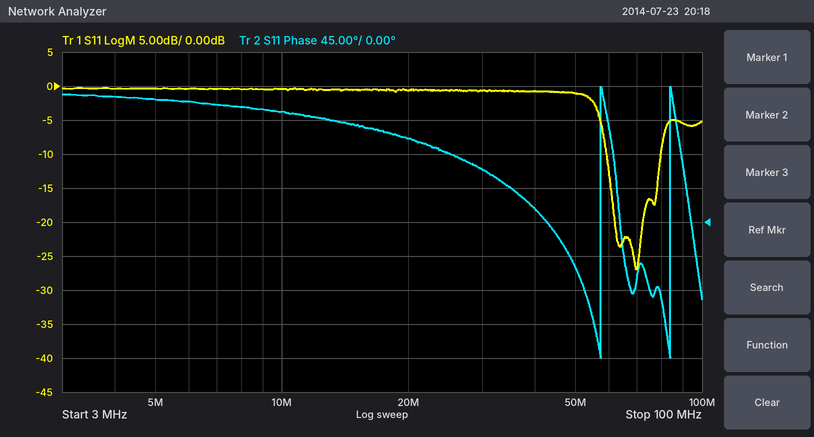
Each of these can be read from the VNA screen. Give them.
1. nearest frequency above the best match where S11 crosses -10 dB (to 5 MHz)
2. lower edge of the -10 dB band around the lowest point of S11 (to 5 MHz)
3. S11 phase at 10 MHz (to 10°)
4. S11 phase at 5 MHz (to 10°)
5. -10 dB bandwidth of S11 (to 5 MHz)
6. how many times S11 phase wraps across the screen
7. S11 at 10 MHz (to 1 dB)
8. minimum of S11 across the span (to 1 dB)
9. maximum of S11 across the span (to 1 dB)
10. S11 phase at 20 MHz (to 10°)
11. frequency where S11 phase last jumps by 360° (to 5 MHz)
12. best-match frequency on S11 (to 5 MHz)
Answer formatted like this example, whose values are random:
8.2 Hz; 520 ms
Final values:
80 MHz; 60 MHz; 150°; 160°; 20 MHz; 2; 0 dB; -27 dB; 0 dB; 110°; 85 MHz; 70 MHz
